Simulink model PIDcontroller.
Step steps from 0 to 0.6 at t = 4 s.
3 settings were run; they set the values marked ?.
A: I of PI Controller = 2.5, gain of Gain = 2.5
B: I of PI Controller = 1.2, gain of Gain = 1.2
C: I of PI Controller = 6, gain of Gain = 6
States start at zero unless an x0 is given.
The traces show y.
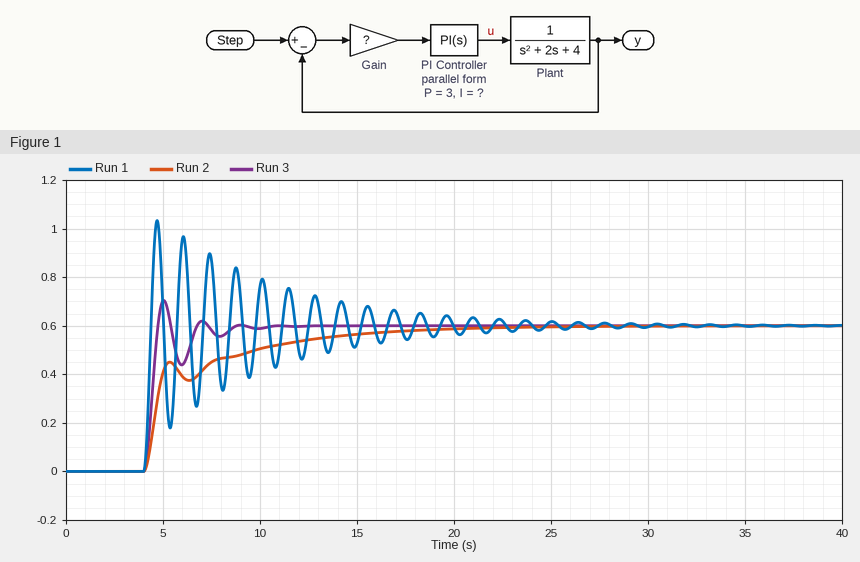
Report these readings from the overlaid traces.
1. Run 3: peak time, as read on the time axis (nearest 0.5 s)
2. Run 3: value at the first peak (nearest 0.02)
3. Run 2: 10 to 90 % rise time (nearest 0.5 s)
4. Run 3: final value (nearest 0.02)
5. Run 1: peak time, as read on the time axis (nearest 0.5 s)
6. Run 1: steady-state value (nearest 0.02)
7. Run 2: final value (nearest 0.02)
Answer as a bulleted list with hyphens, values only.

- 5.0 s
- 0.70
- 8.0 s
- 0.60
- 4.5 s
- 0.60
- 0.60
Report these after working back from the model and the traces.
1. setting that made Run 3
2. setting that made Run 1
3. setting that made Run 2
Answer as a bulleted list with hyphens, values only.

- A
- C
- B
